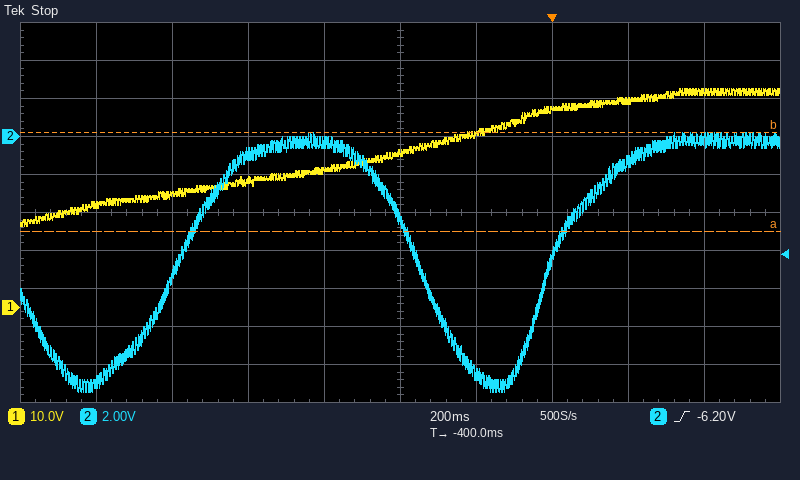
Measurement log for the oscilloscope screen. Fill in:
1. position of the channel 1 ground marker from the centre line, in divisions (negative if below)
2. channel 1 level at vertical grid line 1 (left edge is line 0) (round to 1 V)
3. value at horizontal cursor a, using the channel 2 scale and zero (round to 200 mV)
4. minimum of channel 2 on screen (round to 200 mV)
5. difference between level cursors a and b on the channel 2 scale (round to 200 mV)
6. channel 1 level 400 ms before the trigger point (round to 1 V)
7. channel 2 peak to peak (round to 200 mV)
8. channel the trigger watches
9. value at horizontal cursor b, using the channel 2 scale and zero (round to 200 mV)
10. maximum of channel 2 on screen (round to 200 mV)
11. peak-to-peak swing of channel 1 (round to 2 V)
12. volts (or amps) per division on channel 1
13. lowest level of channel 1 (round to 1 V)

-2.5 div
27 V
-5.0 V
-13.4 V
5.2 V
41 V
13.6 V
channel 2
200 mV
200 mV
36 V
10 V
22 V
